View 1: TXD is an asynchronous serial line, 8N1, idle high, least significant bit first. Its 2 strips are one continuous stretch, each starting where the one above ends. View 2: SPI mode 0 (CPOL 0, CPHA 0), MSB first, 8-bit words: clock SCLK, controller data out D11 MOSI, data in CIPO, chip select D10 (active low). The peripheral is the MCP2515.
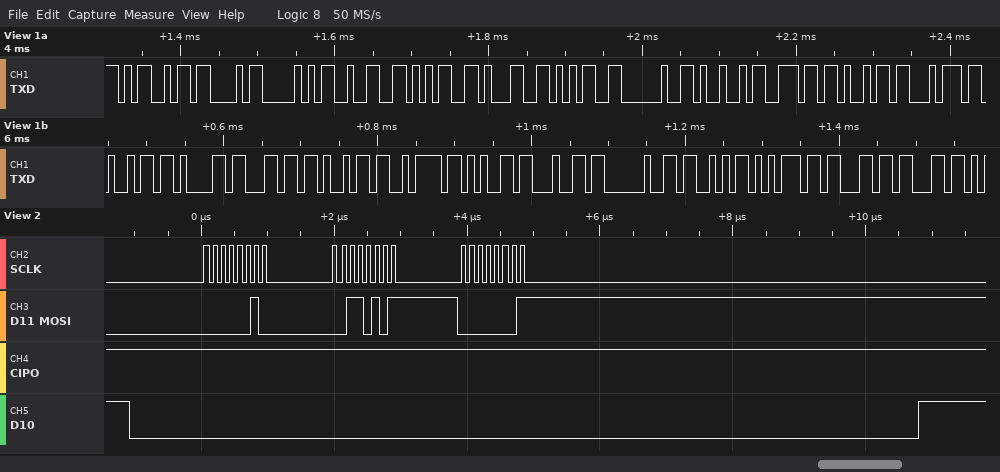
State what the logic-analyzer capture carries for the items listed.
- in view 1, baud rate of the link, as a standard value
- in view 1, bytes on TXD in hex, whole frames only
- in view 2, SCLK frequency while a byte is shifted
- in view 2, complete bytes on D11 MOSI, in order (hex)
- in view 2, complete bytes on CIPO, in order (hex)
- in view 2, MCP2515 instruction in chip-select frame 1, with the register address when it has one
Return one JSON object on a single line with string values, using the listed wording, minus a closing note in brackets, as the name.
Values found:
{"in view 1, baud rate of the link, as a standard value": "115200 baud", "in view 1, bytes on TXD in hex, whole frames only": "4D 43 50 32 35 31 35 20 49 6E 69 74 69 61 6C 69 7A 65 64 20 53 75 63 63", "in view 2, SCLK frequency while a byte is shifted": "8 MHz", "in view 2, complete bytes on D11 MOSI, in order": "02 35 01", "in view 2, complete bytes on CIPO, in order": "FF FF FF", "in view 2, MCP2515 instruction in chip-select frame 1, with the register address when it has one": "WRITE 0x35"}
